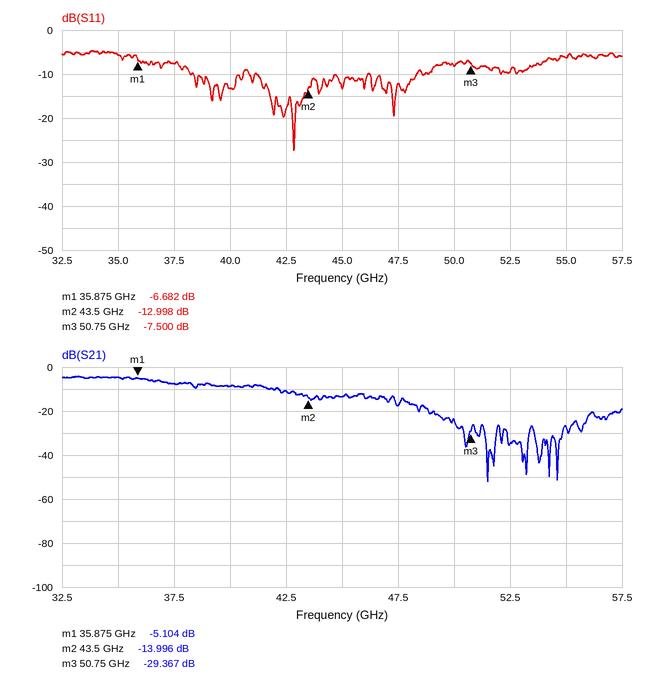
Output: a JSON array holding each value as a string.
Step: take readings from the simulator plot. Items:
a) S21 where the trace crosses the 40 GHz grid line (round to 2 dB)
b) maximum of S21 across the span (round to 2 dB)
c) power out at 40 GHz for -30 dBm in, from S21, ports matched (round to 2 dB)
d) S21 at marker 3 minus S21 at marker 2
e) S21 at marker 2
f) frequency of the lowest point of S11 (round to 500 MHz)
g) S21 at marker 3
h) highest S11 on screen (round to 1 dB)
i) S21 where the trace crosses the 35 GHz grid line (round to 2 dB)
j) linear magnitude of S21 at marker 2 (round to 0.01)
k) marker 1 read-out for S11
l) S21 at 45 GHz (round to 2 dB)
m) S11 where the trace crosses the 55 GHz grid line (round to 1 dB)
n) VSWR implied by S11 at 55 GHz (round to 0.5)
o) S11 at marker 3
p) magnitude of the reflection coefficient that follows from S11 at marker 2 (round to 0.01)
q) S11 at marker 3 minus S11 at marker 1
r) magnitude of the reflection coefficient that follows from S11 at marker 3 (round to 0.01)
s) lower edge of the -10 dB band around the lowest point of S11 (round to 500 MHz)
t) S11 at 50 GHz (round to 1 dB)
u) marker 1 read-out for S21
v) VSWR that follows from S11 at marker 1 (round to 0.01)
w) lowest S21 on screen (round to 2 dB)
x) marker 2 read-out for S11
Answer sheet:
["-8 dB", "-4 dB", "-38 dBm", "-15.371 dB", "-13.996 dB", "43.0 GHz", "-29.367 dB", "-5 dB", "-4 dB", "0.20", "-6.682 dB", "-14 dB", "-6 dB", "3.0", "-7.500 dB", "0.22", "-0.818 dB", "0.42", "41.0 GHz", "-8 dB", "-5.104 dB", "2.73", "-52 dB", "-12.998 dB"]
